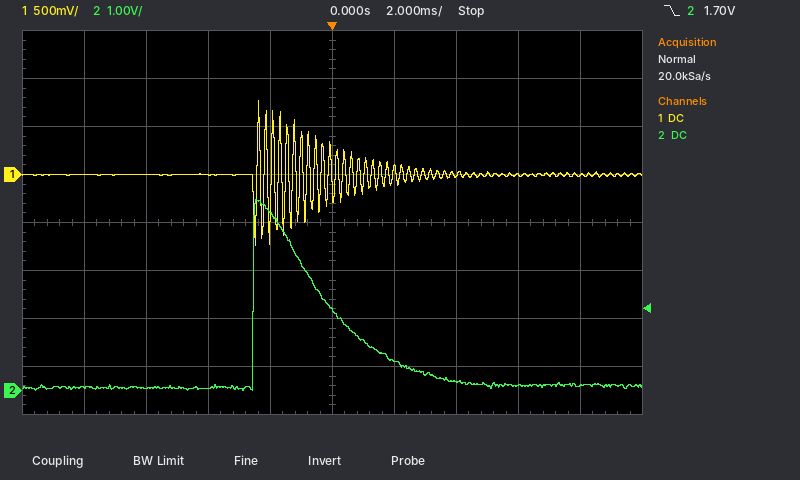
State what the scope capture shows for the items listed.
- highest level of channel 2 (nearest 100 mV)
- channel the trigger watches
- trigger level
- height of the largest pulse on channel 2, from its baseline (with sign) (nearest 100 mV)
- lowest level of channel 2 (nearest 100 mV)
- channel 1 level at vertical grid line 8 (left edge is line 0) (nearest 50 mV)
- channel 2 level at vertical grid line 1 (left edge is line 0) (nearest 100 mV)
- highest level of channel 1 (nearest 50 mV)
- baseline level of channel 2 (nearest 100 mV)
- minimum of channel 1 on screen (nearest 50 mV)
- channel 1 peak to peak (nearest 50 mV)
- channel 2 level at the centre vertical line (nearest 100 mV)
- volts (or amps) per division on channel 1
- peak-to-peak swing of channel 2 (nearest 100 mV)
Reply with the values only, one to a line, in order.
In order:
4.0 V
channel 2
1.70 V
+3.9 V
0.0 V
0 mV
100 mV
750 mV
100 mV
-750 mV
1.50 V
1.7 V
500 mV
4.0 V
